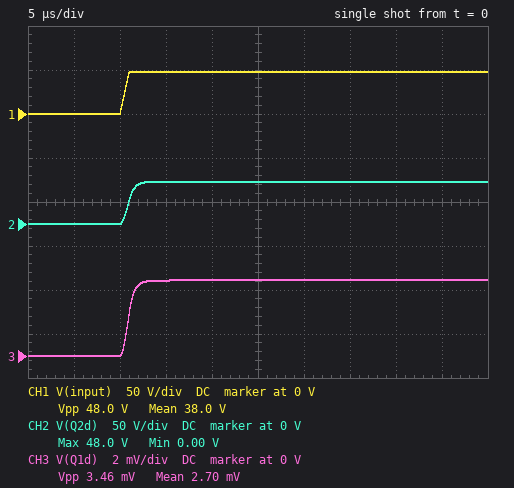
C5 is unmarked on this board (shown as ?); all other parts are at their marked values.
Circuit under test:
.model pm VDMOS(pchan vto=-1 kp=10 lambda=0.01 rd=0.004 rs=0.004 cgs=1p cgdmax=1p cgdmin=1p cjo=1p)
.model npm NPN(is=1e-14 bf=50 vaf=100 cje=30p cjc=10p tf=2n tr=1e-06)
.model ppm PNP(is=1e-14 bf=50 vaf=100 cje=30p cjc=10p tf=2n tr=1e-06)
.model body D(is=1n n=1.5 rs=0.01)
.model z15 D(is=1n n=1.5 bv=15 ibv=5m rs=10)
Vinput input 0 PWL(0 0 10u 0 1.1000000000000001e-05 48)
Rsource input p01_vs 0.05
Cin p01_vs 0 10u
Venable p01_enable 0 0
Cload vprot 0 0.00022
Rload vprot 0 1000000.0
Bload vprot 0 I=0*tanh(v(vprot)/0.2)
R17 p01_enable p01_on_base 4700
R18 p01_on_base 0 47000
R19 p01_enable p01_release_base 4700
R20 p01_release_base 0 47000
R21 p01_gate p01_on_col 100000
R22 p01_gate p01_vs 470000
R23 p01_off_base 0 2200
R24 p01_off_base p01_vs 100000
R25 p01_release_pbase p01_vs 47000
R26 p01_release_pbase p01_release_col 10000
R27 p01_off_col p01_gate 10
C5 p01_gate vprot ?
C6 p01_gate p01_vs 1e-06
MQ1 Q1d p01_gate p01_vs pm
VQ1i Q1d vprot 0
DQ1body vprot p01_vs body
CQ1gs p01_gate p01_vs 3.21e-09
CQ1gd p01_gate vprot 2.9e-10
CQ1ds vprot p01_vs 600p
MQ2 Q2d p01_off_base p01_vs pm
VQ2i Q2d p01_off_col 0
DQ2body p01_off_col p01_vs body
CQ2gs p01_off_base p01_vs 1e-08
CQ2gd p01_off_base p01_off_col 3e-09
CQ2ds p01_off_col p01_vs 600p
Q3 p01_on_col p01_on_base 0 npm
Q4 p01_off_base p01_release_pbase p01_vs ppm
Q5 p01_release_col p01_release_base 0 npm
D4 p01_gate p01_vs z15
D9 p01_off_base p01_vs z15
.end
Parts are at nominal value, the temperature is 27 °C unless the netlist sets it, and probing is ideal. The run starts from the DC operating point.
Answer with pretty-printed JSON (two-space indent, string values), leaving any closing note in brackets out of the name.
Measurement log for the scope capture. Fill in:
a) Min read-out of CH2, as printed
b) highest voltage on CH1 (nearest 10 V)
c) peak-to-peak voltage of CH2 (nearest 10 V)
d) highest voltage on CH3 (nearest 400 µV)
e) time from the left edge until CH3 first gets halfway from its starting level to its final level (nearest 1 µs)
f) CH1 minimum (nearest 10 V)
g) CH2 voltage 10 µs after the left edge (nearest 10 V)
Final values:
{
  "Min read-out of CH2, as printed": "0.00 V",
  "highest voltage on CH1": "50 V",
  "peak-to-peak voltage of CH2": "50 V",
  "highest voltage on CH3": "3.6 mV",
  "time from the left edge until CH3 first gets halfway from its starting level to its final level": "11 µs",
  "CH1 minimum": "0 V",
  "CH2 voltage 10 µs after the left edge": "0 V"
}
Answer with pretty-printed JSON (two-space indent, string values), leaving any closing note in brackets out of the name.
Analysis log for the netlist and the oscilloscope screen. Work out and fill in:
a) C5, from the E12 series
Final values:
{
  "C5, from the E12 series": "15 nF"
}
